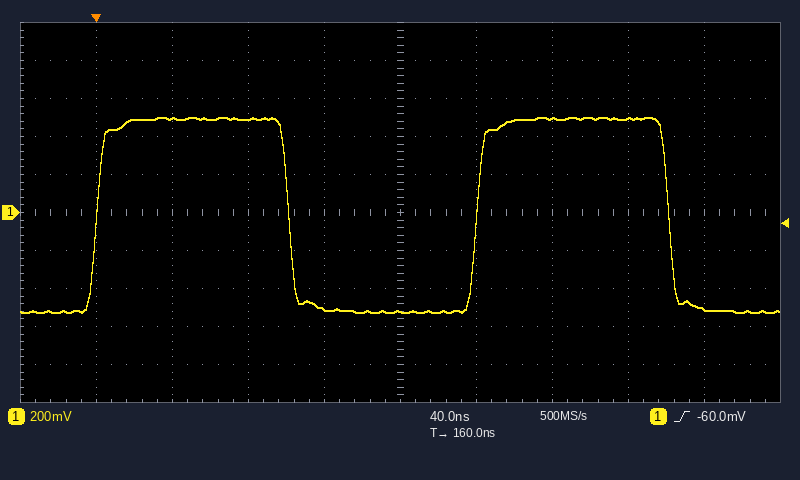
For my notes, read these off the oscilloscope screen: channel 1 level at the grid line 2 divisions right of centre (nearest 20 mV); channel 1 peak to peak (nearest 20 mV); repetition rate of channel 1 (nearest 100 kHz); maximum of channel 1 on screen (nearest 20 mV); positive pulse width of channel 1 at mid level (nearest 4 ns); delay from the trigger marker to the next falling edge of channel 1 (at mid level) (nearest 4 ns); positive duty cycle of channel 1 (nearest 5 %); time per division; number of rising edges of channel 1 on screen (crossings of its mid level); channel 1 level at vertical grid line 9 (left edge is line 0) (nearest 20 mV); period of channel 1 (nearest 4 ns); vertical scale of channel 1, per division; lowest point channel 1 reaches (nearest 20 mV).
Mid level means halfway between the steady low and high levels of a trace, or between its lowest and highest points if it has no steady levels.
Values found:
500 mV
1.02 V
5.0 MHz
500 mV
100 ns
100 ns
50 %
40 ns
2
-500 mV
200 ns
200 mV
-520 mV
